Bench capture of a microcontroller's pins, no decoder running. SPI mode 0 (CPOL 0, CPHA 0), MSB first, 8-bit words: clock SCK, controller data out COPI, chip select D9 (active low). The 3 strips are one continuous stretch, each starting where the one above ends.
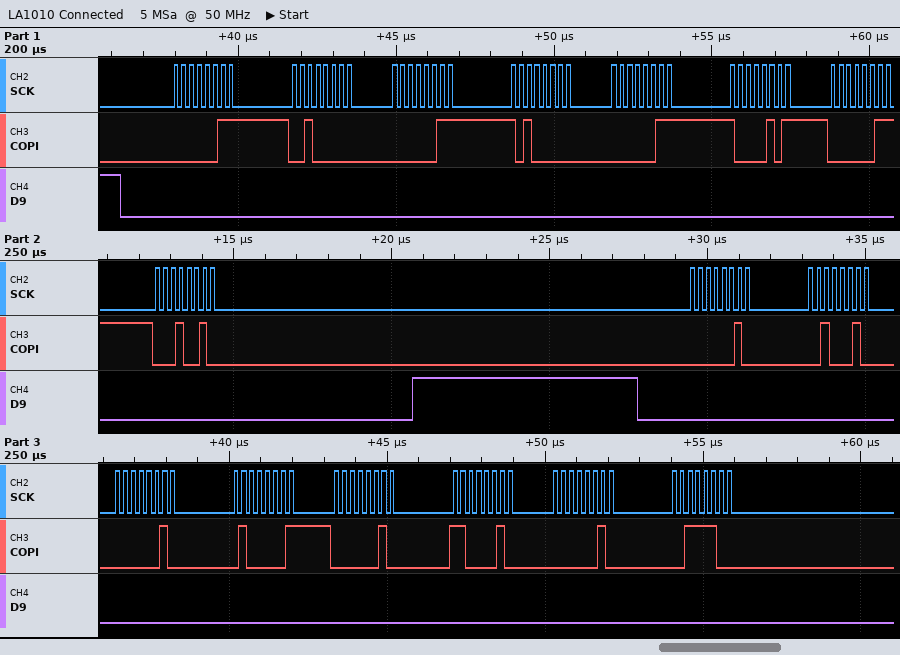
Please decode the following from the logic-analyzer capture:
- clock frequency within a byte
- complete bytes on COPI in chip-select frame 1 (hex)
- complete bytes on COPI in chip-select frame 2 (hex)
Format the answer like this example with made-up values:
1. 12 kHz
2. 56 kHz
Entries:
1. 4 MHz
2. 03 20 03 A0 03 85 03 12
3. 02 22 02 41 02 C2 02 3C
